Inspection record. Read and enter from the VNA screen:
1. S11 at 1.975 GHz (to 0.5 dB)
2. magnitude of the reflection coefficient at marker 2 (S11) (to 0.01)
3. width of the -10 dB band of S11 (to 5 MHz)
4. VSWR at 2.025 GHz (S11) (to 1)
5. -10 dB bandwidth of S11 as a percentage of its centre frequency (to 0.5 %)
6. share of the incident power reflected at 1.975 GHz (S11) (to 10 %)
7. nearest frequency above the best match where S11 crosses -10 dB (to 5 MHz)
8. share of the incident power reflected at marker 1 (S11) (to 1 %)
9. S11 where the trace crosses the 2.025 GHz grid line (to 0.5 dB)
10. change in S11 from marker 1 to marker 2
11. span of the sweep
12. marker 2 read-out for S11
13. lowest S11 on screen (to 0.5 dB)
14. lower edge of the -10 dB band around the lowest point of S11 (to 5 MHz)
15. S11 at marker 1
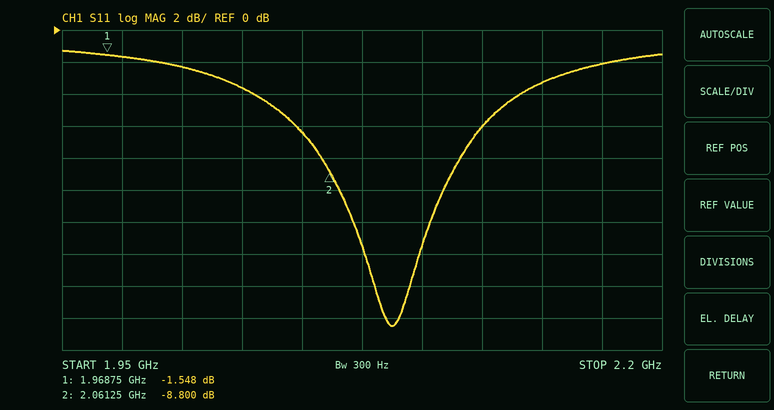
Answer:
-1.5 dB
0.36
45 MHz
5
2.0 %
70 %
2.110 GHz
70 %
-3.5 dB
-7.252 dB
250 MHz
-8.800 dB
-18.5 dB
2.065 GHz
-1.548 dB
